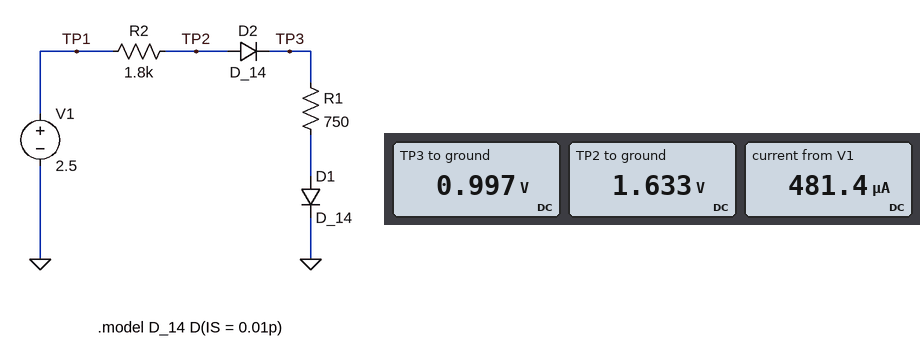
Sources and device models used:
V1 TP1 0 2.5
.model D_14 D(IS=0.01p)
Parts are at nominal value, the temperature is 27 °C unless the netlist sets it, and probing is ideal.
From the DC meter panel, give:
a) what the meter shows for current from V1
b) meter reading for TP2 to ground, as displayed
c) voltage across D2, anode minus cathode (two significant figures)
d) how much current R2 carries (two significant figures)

481.4 µA
1.633 V
640 mV
480 µA
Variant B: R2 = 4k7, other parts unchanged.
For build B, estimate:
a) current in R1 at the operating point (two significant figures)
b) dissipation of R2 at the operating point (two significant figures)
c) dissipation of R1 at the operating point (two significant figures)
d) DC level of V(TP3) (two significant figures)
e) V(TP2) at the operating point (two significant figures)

230 µA
250 µW
40 µW
790 mV
1.4 V
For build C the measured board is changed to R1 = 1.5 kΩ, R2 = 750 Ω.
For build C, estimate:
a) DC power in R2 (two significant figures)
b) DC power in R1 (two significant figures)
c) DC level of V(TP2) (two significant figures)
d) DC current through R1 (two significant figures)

220 µW
440 µW
2.1 V
540 µA
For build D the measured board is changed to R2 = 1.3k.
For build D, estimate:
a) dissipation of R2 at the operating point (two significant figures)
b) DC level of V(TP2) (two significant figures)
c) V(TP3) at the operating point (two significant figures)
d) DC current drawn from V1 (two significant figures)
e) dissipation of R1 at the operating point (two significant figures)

460 µW
1.7 V
1.1 V
590 µA
260 µW
